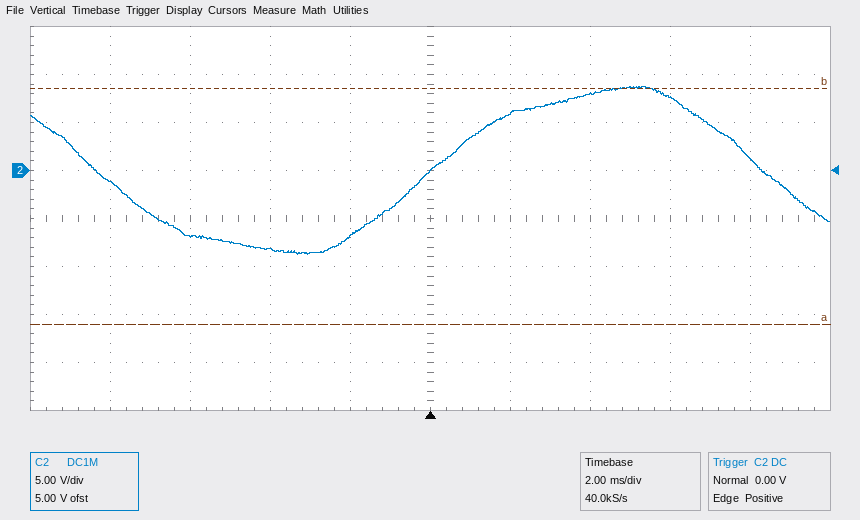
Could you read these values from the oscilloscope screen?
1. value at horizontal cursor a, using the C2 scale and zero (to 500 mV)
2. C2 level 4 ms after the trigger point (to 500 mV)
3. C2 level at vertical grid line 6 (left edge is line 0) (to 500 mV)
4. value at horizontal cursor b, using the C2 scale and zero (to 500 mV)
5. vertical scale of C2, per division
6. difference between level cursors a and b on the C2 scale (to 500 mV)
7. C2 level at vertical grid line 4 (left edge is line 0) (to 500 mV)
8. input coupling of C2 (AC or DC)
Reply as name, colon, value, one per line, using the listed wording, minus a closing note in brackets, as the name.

value at horizontal cursor a, using the C2 scale and zero: -16.0 V
C2 level 4 ms after the trigger point: 8.0 V
C2 level at vertical grid line 6 (left edge is line 0): 6.0 V
value at horizontal cursor b, using the C2 scale and zero: 8.5 V
vertical scale of C2, per division: 5 V
difference between level cursors a and b on the C2 scale: 24.5 V
C2 level at vertical grid line 4 (left edge is line 0): -7.0 V
input coupling of C2: DC
